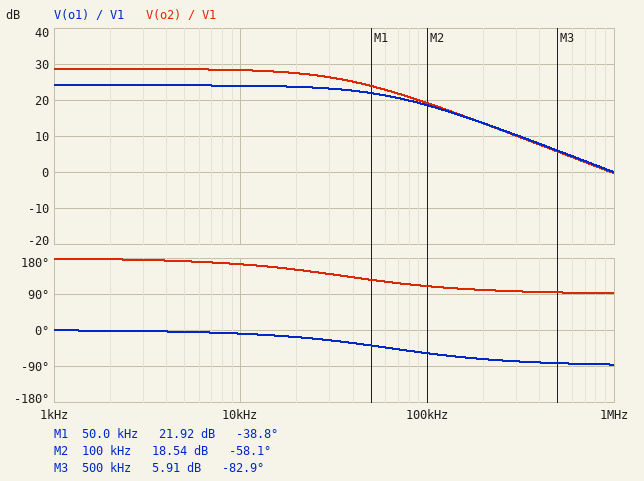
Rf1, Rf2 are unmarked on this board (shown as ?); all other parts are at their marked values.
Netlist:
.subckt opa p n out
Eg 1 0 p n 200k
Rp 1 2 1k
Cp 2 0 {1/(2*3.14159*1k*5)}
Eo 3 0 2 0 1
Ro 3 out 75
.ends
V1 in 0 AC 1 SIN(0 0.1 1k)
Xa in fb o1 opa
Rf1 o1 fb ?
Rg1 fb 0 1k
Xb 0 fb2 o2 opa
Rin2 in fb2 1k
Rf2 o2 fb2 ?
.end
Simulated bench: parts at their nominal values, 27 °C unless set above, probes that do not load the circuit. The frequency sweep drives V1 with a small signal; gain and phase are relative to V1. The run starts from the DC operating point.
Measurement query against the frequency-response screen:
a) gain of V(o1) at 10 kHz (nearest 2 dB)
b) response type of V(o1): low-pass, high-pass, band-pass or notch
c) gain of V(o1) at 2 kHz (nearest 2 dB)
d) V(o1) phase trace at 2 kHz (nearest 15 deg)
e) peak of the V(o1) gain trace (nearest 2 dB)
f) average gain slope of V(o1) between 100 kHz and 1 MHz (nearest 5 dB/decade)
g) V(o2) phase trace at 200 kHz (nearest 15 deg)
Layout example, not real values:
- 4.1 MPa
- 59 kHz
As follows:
- 24 dB
- low-pass
- 24 dB
- 0 deg
- 24 dB
- -20 dB/decade
- 105 deg
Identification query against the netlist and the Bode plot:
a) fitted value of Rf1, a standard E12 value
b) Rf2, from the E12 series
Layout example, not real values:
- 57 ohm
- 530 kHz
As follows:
- 15 kΩ
- 27 kΩ
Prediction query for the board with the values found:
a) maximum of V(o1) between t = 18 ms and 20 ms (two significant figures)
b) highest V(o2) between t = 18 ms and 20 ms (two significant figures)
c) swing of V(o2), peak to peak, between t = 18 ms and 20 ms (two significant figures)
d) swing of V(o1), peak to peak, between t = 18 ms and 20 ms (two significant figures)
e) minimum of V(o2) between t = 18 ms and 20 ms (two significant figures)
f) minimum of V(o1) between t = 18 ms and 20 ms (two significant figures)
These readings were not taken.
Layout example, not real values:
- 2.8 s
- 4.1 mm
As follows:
- 1.6 V
- 2.7 V
- 5.4 V
- 3.2 V
- -2.7 V
- -1.6 V
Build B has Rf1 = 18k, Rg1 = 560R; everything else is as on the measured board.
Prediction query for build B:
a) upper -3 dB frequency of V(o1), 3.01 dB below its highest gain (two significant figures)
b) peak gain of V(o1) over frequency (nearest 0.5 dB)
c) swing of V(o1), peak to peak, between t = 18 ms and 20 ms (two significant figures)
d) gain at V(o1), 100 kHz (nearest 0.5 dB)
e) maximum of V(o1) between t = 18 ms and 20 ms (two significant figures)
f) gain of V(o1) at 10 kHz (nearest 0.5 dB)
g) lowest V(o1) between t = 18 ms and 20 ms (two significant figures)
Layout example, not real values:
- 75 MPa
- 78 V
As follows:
- 30 kHz
- 30.5 dB
- 6.6 V
- 19.5 dB
- 3.3 V
- 30.0 dB
- -3.3 V
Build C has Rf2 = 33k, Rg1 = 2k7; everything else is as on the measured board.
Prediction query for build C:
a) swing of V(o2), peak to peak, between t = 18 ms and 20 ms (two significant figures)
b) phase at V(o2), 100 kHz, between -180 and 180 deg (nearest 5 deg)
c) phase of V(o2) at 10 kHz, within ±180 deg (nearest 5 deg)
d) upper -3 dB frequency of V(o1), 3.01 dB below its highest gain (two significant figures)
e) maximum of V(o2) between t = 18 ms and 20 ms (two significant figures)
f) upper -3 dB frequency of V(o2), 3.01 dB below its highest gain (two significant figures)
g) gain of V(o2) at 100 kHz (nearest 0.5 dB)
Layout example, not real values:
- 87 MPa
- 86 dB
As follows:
- 6.6 V
- 105 deg
- 160 deg
- 150 kHz
- 3.3 V
- 29 kHz
- 19.5 dB
